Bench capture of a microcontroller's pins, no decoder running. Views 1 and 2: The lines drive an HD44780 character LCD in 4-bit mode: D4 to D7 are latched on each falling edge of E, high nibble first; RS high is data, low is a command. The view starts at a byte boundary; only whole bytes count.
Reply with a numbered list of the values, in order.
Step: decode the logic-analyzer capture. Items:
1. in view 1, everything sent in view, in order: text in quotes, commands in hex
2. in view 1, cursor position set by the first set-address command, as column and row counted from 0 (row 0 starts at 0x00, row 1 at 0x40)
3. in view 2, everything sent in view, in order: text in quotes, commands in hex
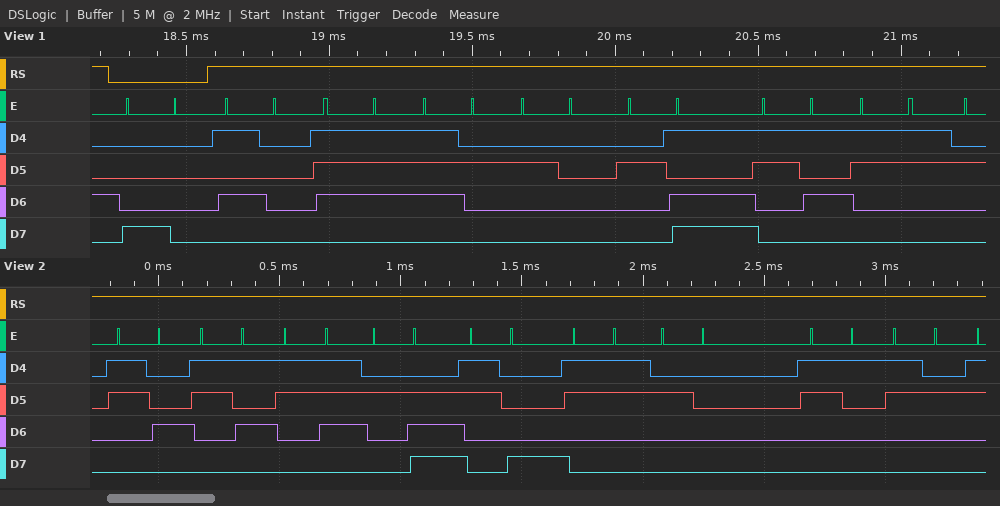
1. 0x80 "Pwr -53"
2. column 0, row 0
3. "457.83 12"
